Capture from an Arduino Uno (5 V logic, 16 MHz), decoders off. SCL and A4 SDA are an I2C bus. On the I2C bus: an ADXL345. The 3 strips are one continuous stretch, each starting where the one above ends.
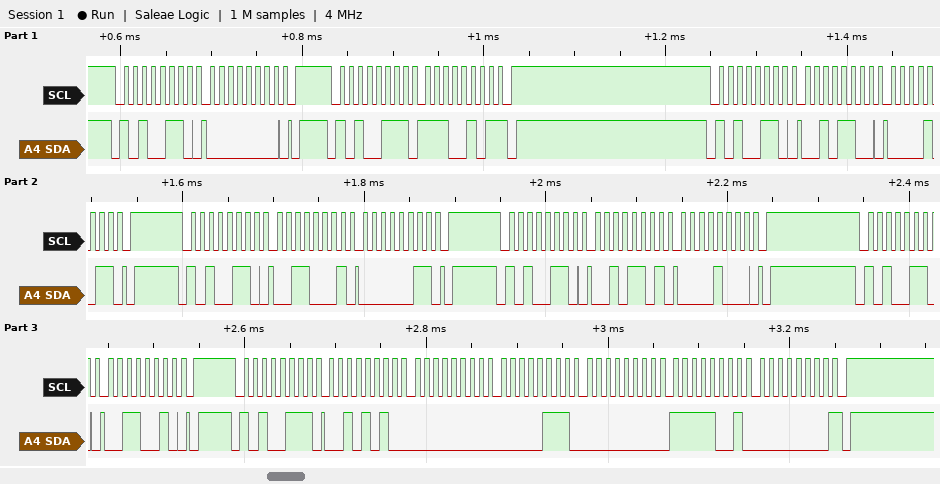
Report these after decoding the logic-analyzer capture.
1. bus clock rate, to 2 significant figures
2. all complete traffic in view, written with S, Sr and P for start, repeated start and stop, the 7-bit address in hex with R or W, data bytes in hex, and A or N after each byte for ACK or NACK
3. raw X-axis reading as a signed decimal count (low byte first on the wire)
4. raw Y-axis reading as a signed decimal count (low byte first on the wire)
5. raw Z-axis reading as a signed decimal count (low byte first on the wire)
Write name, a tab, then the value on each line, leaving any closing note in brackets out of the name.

bus clock rate, to 2 significant figures	100 kHz
all complete traffic in view, written with S, Sr and P for start, repeated start and stop, the 7-bit address in hex with R or W, data bytes in hex, and A or N after each byte for ACK or NACK	S 53W A 00 A P S 53R A E5 N P S 53W A 2C A 0B A P S 53W A 31 A 03 A P S 53W A 2D A 08 A P S 53W A 32 A P S 53R A 2A A 00 A 07 A 00 A F9 A 00 N P
raw X-axis reading as a signed decimal count	42
raw Y-axis reading as a signed decimal count	7
raw Z-axis reading as a signed decimal count	249
